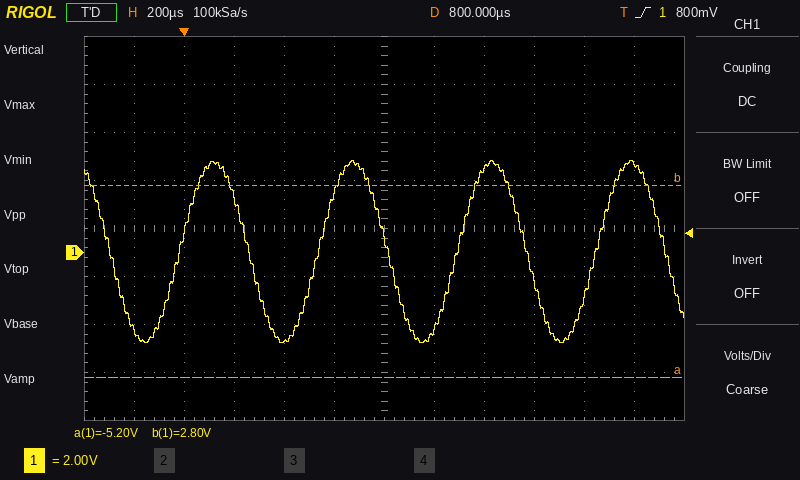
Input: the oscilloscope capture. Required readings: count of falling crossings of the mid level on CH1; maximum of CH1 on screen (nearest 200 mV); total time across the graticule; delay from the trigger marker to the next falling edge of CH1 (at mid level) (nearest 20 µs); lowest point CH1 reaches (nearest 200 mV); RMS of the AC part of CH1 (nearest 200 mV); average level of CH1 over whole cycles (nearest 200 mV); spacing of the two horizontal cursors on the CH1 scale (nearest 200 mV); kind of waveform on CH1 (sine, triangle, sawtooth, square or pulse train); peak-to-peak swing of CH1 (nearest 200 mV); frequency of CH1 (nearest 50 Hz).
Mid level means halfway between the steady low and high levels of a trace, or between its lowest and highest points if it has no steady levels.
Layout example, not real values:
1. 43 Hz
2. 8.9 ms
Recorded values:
1. 5
2. 3.8 V
3. 2.4 ms
4. 260 µs
5. -3.8 V
6. 2.6 V
7. 0.0 V
8. 8.0 V
9. sine
10. 7.6 V
11. 1.80 kHz
